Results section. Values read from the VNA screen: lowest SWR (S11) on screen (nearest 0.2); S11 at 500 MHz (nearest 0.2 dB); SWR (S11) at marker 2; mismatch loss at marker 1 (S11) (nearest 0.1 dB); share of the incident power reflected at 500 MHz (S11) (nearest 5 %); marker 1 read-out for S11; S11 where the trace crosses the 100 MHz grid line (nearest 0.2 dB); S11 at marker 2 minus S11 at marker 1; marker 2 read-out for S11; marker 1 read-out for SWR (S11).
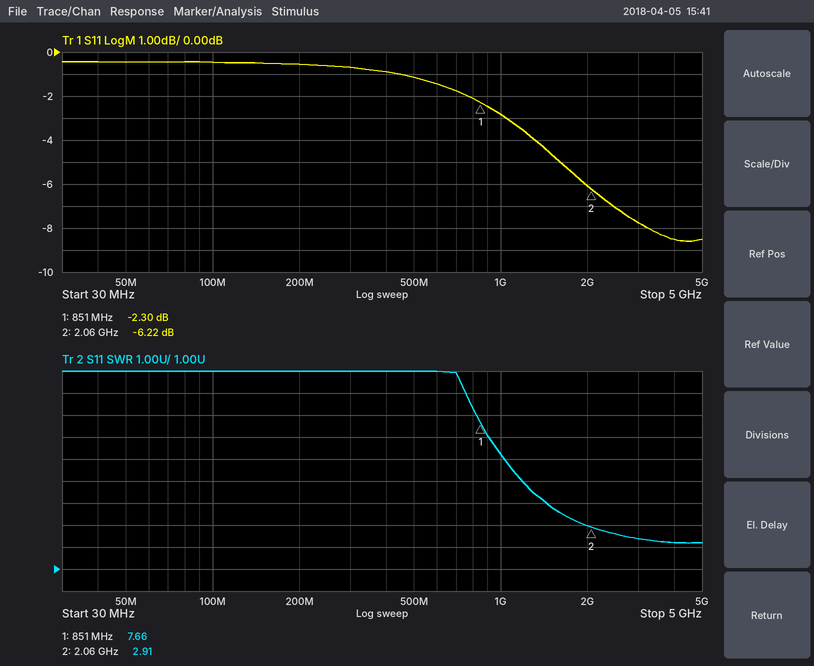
2.2
-1.2 dB
2.91
3.9 dB
75 %
-2.30 dB
-0.4 dB
-3.92 dB
-6.22 dB
7.66
